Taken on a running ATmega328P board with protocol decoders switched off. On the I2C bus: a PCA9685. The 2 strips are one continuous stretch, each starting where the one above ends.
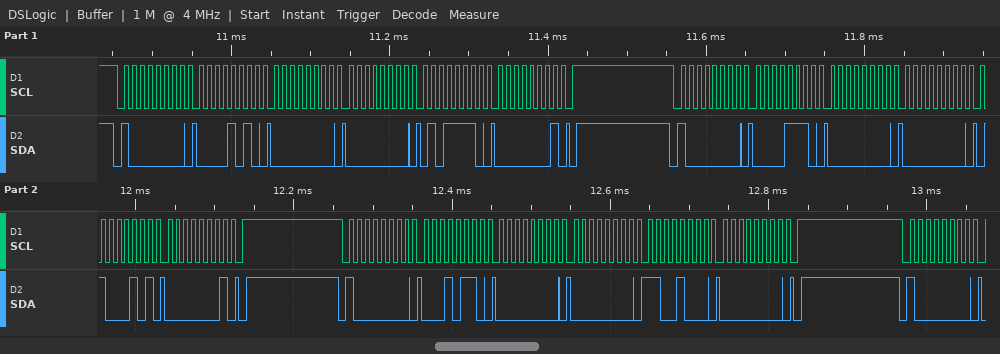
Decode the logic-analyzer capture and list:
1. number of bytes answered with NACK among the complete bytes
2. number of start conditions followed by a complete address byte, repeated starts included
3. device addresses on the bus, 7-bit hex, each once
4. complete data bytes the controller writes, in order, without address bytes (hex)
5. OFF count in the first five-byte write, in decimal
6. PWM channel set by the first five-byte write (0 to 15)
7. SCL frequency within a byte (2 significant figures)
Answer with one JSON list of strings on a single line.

["0", "4", "0x40", "0A 00 00 5E 01 0E 00 00 45 01 16 00 00 C8 00", "350", "1", "100 kHz"]
